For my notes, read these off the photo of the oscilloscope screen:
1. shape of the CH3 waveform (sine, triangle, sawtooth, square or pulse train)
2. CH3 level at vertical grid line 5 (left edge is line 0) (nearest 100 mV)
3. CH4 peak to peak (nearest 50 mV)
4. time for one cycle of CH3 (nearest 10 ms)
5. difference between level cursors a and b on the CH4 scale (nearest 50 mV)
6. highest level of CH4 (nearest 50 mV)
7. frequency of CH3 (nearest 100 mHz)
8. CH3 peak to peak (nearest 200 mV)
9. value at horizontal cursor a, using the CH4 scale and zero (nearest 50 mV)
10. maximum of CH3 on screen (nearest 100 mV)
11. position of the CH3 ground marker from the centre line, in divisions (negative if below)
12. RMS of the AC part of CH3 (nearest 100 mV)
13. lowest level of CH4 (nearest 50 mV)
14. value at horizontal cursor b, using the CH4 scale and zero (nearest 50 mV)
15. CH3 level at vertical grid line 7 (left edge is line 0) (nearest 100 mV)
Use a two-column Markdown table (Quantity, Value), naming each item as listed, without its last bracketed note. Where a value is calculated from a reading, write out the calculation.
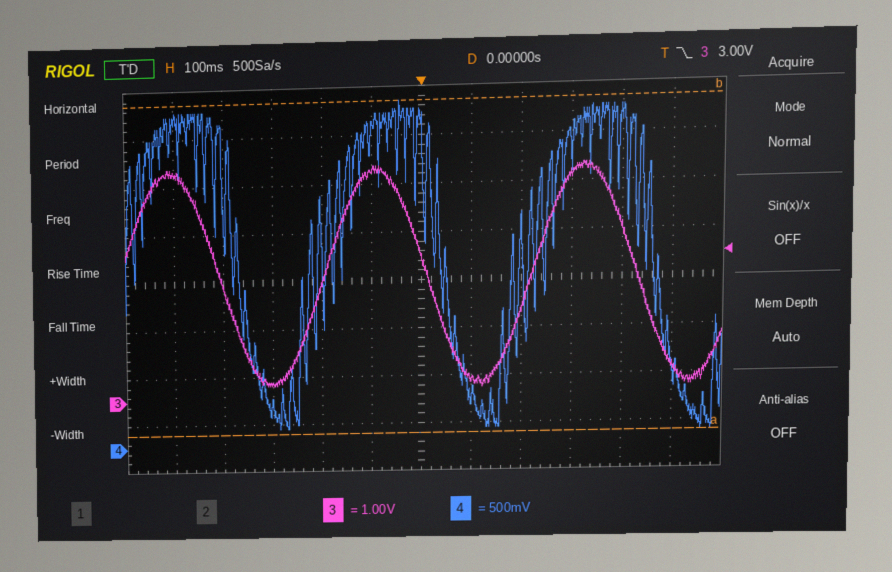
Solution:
| Quantity | Value |
|---|---|
| shape of the CH3 waveform | sine |
| CH3 level at vertical grid line 5 (left edge is line 0) | 4.8 V |
| CH4 peak to peak | 3.60 V − (150 mV) = 3.45 V |
| time for one cycle of CH3 | 420 ms |
| difference between level cursors a and b on the CH4 scale | 3.45 V |
| highest level of CH4 | 3.60 V |
| frequency of CH3 | 1 / 420 ms ≈ 2.4 Hz |
| CH3 peak to peak | 4.6 V |
| value at horizontal cursor a, using the CH4 scale and zero | 150 mV |
| maximum of CH3 on screen | 4.9 V |
| position of the CH3 ground marker from the centre line, in divisions | -2.5 div |
| RMS of the AC part of CH3 | 4.6 V / (2√2) ≈ 1.6 V |
| lowest level of CH4 | 150 mV |
| value at horizontal cursor b, using the CH4 scale and zero | 3.60 V |
| CH3 level at vertical grid line 7 (left edge is line 0) | 400 mV |
